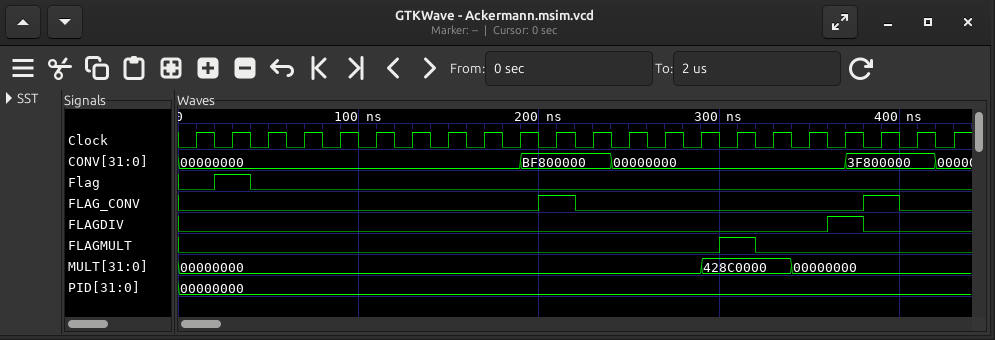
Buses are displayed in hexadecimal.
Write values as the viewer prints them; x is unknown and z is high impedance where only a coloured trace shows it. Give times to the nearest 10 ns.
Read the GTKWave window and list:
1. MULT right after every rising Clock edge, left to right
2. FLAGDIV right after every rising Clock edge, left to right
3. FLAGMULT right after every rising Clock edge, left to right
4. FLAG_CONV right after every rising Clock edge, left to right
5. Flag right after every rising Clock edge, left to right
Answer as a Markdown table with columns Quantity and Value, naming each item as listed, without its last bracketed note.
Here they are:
| Quantity | Value |
|---|---|
| MULT right after every rising Clock edge, left to right | 00000000, 00000000, 00000000, 00000000, 00000000, 00000000, 00000000, 00000000, 00000000, 00000000, 00000000, 00000000, 00000000, 00000000, 428C0000, 428C0000, 428C0000, 00000000, 00000000, 00000000, 00000000, 00000000 |
| FLAGDIV right after every rising Clock edge, left to right | 0 0 0 0 0 0 0 0 0 0 0 0 0 0 0 0 0 0 1 0 0 0 |
| FLAGMULT right after every rising Clock edge, left to right | 0 0 0 0 0 0 0 0 0 0 0 0 0 0 0 1 0 0 0 0 0 0 |
| FLAG_CONV right after every rising Clock edge, left to right | 0 0 0 0 0 0 0 0 0 0 1 0 0 0 0 0 0 0 0 1 0 0 |
| Flag right after every rising Clock edge, left to right | 0 1 0 0 0 0 0 0 0 0 0 0 0 0 0 0 0 0 0 0 0 0 |
